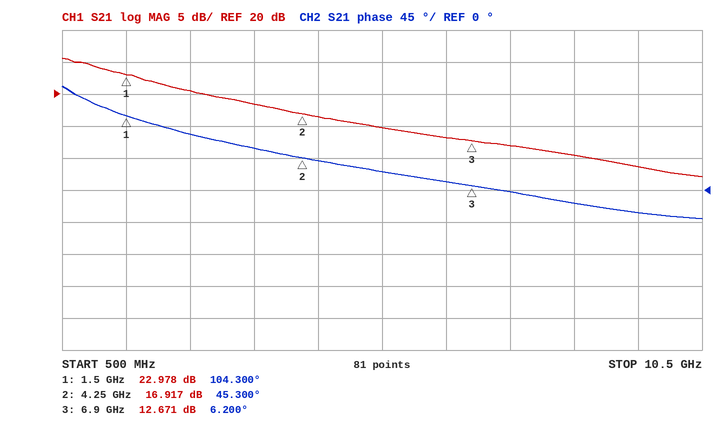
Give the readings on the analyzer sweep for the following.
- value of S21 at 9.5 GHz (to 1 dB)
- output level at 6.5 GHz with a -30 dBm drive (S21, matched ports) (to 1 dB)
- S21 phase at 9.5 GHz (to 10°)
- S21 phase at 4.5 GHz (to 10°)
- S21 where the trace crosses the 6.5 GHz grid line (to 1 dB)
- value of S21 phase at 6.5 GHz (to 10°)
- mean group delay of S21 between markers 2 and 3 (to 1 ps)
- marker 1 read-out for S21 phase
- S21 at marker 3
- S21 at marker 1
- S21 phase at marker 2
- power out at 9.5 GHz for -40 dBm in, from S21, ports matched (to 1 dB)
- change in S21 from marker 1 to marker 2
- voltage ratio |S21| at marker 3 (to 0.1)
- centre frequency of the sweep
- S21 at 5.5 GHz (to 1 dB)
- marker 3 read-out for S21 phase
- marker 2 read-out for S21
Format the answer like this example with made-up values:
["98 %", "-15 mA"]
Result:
["9 dB", "-17 dBm", "-30°", "40°", "13 dB", "10°", "41 ps", "104.300°", "12.671 dB", "22.978 dB", "45.300°", "-31 dBm", "-6.061 dB", "4.3", "5.5 GHz", "15 dB", "6.200°", "16.917 dB"]
